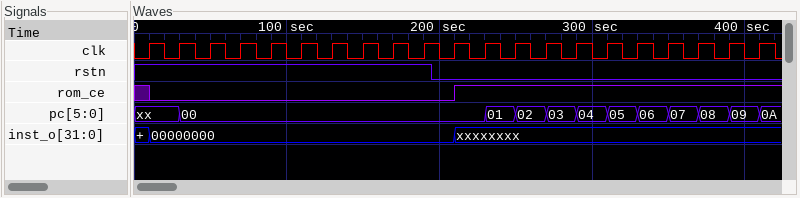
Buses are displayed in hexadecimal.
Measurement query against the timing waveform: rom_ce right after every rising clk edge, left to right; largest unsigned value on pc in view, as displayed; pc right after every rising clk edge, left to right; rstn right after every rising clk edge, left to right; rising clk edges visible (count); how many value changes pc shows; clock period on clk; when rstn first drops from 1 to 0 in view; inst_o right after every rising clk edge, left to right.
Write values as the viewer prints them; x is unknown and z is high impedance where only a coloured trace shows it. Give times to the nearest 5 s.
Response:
0 0 0 0 0 0 0 0 0 0 1 1 1 1 1 1 1 1 1 1 1
0A
xx, 00, 00, 00, 00, 00, 00, 00, 00, 00, 00, 01, 02, 03, 04, 05, 06, 07, 08, 09, 0A
1 1 1 1 1 1 1 1 1 1 0 0 0 0 0 0 0 0 0 0 0
21
11
20 s
195 s
00000000, 00000000, 00000000, 00000000, 00000000, 00000000, 00000000, 00000000, 00000000, 00000000, xxxxxxxx, xxxxxxxx, xxxxxxxx, xxxxxxxx, xxxxxxxx, xxxxxxxx, xxxxxxxx, xxxxxxxx, xxxxxxxx, xxxxxxxx, xxxxxxxx
